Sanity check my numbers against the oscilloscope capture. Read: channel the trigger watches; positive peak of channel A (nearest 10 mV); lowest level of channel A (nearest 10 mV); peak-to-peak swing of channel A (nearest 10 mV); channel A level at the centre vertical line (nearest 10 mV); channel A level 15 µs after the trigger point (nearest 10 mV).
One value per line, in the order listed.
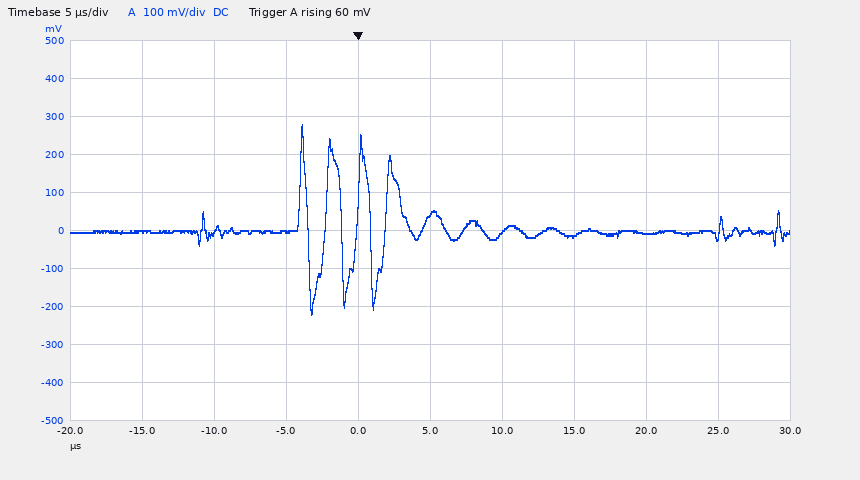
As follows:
channel A
280 mV
-220 mV
500 mV
40 mV
-10 mV
